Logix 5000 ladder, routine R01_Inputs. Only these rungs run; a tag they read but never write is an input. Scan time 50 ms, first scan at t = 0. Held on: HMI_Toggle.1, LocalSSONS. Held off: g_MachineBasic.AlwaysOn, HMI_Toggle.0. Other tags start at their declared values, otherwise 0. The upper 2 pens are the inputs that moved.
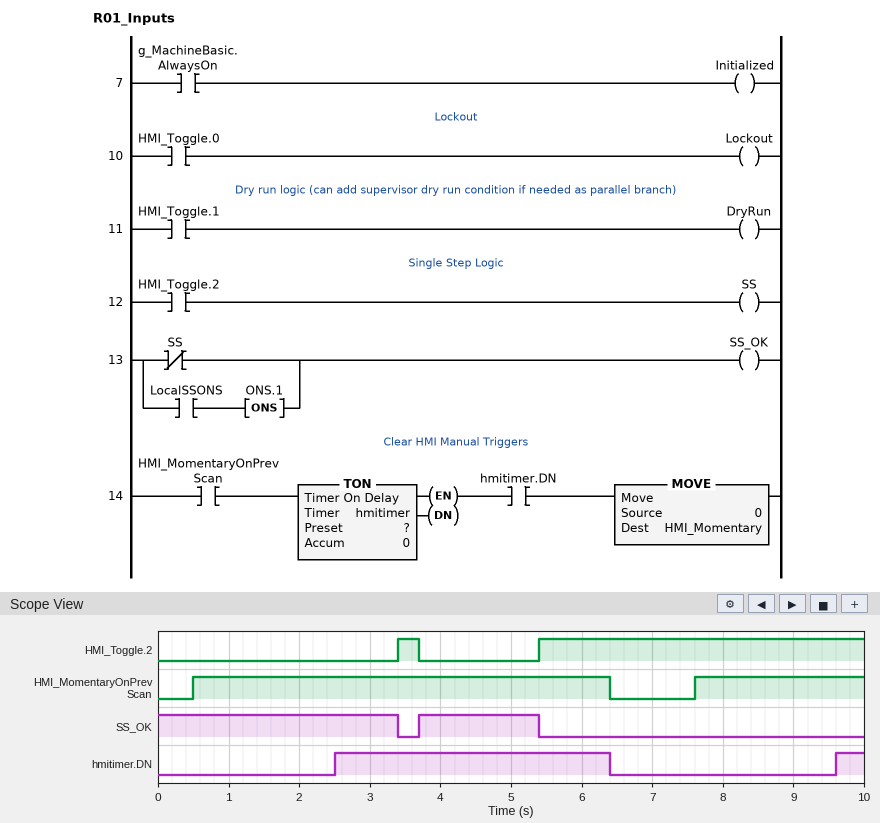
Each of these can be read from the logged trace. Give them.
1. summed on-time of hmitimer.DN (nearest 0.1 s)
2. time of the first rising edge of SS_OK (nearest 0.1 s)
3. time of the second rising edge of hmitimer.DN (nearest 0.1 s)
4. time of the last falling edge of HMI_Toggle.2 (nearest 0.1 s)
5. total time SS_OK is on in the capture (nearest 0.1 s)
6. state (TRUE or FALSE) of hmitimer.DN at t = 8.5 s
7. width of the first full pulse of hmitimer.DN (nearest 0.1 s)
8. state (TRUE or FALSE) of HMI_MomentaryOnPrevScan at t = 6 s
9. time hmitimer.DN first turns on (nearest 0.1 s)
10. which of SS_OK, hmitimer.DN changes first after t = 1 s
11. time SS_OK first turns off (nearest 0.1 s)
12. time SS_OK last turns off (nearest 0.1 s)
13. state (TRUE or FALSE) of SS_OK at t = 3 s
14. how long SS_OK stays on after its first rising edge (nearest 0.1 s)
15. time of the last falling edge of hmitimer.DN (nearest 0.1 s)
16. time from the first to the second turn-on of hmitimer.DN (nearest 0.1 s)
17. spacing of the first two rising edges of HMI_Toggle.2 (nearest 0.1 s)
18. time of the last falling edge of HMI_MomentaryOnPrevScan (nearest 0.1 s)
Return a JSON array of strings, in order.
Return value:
["4.3 s", "3.7 s", "9.6 s", "3.7 s", "5.1 s", "FALSE", "3.9 s", "TRUE", "2.5 s", "hmitimer.DN", "3.4 s", "5.4 s", "TRUE", "1.7 s", "6.4 s", "7.1 s", "2.0 s", "6.4 s"]
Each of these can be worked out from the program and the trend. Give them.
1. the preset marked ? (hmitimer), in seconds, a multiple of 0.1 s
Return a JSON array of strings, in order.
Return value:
["2.0 s"]
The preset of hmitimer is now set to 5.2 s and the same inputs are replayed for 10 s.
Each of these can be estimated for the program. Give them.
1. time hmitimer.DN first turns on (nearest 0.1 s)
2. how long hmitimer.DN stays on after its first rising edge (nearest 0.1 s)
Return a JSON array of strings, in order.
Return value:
["5.7 s", "0.7 s"]
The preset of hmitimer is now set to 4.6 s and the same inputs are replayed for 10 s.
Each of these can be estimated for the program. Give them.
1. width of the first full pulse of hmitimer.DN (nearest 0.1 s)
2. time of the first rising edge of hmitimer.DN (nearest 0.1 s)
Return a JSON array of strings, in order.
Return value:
["1.3 s", "5.1 s"]
